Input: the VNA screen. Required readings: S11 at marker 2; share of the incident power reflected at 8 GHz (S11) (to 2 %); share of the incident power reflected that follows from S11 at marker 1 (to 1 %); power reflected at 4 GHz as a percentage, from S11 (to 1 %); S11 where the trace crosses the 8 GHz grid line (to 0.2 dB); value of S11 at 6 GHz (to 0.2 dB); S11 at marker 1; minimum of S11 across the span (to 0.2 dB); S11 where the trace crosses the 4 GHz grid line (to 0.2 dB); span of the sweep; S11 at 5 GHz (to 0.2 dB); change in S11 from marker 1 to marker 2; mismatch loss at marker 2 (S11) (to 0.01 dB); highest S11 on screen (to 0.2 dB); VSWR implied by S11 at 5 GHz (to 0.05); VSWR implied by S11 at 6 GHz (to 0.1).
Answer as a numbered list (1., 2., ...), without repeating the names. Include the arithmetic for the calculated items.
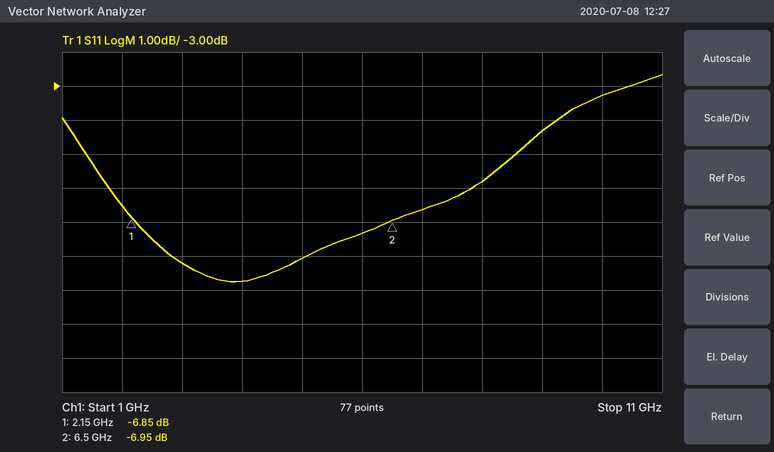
1. -6.95 dB
2. 10^(-5.8/10) ≈ 26 %
3. 10^(-6.85/10) ≈ 21 %
4. 10^(-8.8/10) ≈ 13 %
5. -5.8 dB
6. -7.4 dB
7. -6.85 dB
8. -8.8 dB
9. -8.8 dB
10. 10 GHz
11. -8.0 dB
12. -6.95 − (-6.85) = -0.10 dB
13. −10 log10(1 − 10^(-6.95/10)) ≈ 0.98 dB
14. -2.6 dB
15. |Γ| = 10^(-8/20) = 0.3981; VSWR = (1 + 0.3981)/(1 − 0.3981) ≈ 2.32, so 2.30 to the nearest 0.05
16. |Γ| = 10^(-7.4/20) = 0.4266; VSWR = (1 + 0.4266)/(1 − 0.4266) ≈ 2.5
